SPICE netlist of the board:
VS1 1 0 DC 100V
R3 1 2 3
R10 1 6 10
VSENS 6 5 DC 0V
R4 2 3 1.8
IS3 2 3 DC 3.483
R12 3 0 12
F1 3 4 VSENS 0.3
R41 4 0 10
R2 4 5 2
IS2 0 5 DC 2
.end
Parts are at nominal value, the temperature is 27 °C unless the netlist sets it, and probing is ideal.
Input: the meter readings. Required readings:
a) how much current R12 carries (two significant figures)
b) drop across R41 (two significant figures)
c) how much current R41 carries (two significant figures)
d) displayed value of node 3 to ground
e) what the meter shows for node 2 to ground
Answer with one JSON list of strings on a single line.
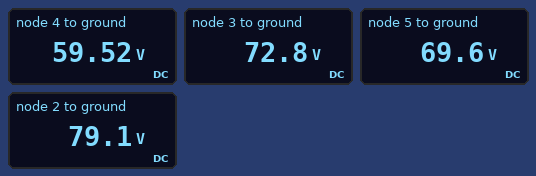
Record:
["6.1 A", "60 V", "6.0 A", "72.8 V", "79.1 V"]
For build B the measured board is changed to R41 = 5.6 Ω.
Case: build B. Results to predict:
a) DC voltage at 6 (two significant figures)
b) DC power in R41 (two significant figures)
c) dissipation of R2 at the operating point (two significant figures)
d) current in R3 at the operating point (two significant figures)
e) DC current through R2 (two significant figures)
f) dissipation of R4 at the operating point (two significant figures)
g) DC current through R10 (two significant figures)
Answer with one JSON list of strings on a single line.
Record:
["56 V", "330 W", "82 W", "7.3 A", "6.4 A", "26 W", "4.4 A"]
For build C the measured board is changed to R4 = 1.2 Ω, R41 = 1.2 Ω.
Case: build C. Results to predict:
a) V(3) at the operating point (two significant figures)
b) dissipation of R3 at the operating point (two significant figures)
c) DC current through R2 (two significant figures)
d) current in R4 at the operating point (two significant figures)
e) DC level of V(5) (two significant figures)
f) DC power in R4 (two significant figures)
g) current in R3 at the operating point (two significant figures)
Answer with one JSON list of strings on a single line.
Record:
["71 V", "190 W", "8.9 A", "4.5 A", "31 V", "24 W", "8.0 A"]
